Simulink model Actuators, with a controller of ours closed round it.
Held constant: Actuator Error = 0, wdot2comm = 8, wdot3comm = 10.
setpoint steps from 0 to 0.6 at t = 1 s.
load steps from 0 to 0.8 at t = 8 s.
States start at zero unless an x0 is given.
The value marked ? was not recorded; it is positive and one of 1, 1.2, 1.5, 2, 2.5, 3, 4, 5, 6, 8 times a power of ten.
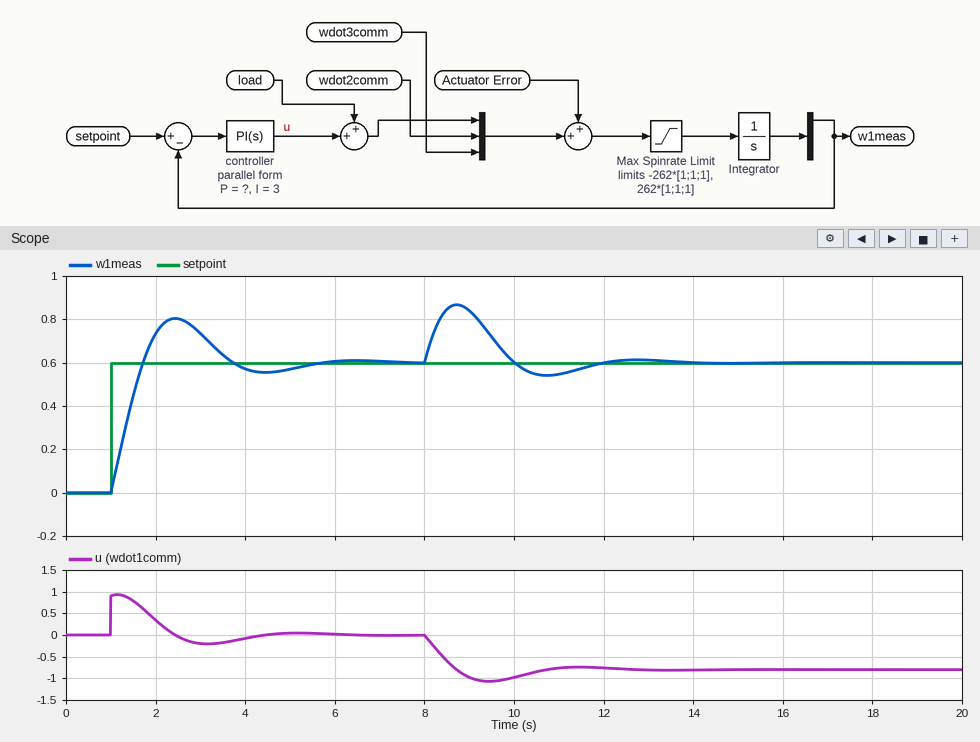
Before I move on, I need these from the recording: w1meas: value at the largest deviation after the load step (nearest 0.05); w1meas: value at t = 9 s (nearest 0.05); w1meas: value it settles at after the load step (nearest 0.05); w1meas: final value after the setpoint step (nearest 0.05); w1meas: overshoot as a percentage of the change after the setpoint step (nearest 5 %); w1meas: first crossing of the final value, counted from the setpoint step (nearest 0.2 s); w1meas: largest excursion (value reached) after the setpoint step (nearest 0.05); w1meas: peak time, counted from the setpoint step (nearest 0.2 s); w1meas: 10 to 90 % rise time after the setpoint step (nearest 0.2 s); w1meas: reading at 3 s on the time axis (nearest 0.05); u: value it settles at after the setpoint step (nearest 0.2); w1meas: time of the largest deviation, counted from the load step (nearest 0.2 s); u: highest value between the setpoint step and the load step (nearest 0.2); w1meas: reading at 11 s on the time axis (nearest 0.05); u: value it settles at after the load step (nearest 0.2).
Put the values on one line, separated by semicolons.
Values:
0.85; 0.85; 0.60; 0.60; 35 %; 0.8 s; 0.80; 1.4 s; 0.6 s; 0.75; 0.0; 0.8 s; 1.0; 0.55; -0.8
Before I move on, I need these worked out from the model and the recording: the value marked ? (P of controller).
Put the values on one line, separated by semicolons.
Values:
1.5
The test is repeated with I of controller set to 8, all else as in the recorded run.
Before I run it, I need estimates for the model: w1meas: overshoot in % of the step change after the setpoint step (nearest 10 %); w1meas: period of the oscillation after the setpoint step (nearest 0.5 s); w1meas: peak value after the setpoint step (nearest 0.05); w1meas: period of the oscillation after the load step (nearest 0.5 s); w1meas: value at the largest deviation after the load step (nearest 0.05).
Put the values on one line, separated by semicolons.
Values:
50 %; 2.5 s; 0.90; 2.5 s; 0.80
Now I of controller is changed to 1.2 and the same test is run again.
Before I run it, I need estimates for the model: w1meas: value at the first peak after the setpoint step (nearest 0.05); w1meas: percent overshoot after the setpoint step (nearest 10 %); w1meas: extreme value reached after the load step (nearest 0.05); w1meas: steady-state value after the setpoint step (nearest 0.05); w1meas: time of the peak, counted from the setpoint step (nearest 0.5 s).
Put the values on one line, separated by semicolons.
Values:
0.75; 20 %; 0.95; 0.60; 2.0 s
